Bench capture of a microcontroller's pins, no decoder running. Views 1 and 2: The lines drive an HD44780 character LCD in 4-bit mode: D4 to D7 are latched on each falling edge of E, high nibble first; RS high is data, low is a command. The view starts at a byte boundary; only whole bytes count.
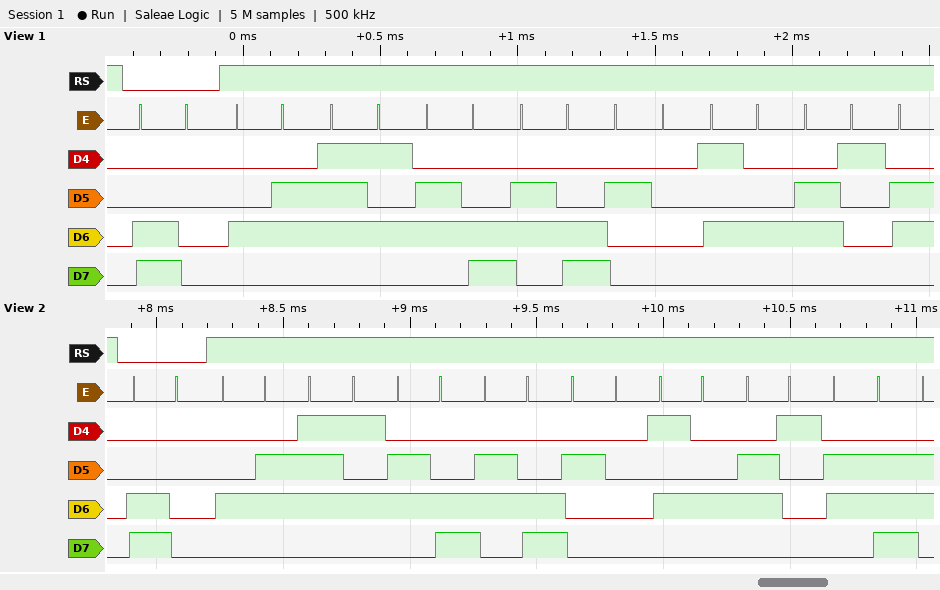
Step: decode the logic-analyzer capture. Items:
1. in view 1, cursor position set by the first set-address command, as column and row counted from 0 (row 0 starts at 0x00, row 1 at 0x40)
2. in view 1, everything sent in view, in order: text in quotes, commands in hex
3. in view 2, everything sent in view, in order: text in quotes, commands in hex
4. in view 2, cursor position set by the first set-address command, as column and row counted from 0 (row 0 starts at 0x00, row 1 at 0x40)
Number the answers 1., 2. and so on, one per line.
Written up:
1. column 0, row 1
2. 0xC0 "Full Ta"
3. 0xC0 "Full Tan"
4. column 0, row 1
